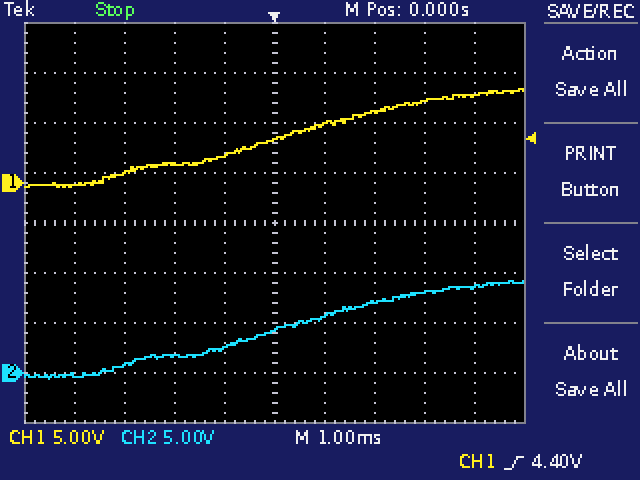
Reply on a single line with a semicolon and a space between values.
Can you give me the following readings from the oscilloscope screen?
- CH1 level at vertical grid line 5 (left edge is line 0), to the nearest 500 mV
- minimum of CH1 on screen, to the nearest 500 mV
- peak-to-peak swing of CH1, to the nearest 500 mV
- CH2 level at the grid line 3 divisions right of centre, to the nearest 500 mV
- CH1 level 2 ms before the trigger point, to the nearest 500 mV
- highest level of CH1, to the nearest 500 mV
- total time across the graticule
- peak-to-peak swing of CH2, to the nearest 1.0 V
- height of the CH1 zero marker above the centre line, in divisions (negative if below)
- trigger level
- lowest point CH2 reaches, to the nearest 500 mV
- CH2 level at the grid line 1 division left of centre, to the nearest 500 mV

4.5 V; -500 mV; 10.0 V; 8.0 V; 2.0 V; 9.5 V; 10 ms; 10.0 V; +0.8 div; 4.40 V; -500 mV; 2.5 V
